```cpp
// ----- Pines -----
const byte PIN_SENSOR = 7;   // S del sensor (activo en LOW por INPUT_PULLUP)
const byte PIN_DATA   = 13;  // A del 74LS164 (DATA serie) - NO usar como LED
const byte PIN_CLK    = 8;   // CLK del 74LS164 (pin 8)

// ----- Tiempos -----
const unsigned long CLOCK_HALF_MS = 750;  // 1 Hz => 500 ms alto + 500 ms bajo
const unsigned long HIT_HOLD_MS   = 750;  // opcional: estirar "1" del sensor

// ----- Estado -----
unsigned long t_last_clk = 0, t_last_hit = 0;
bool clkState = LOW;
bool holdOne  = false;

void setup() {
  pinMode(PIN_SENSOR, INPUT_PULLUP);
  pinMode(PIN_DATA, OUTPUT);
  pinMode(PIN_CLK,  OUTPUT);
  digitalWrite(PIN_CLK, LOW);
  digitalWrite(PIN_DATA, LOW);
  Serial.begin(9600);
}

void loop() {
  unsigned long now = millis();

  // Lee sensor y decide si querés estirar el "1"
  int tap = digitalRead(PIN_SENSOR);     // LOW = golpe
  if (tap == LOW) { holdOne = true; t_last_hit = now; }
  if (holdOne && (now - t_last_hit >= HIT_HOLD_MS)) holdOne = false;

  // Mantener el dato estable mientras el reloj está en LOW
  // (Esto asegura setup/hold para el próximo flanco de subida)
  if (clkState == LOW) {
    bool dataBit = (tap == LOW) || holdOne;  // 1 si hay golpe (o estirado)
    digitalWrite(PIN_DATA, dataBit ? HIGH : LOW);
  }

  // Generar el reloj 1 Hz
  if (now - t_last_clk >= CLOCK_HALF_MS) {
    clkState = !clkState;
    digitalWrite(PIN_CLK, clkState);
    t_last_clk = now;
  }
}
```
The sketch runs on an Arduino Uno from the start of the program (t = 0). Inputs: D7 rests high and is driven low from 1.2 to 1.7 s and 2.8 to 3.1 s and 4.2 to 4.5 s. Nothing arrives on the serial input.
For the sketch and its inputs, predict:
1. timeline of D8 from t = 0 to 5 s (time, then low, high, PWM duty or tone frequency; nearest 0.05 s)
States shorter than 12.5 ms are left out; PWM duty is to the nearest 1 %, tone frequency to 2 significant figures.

0 s low; 0.75 s high; 1.5 s low; 2.25 s high; 3 s low; 3.75 s high; 4.5 s low
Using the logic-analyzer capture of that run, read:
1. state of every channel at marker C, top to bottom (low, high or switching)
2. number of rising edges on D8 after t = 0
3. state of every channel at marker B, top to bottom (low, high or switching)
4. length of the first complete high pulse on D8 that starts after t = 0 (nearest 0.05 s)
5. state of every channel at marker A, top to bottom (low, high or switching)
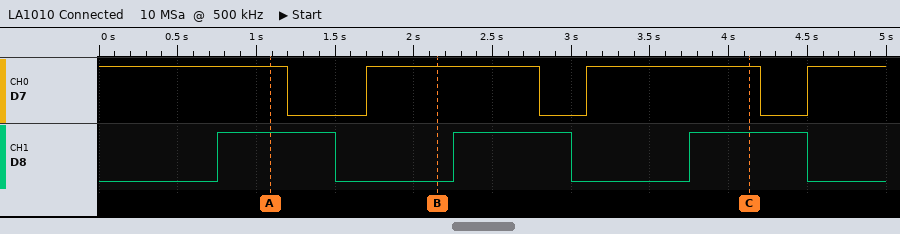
D7 high, D8 high
3
D7 high, D8 low
0.75 s
D7 high, D8 high
